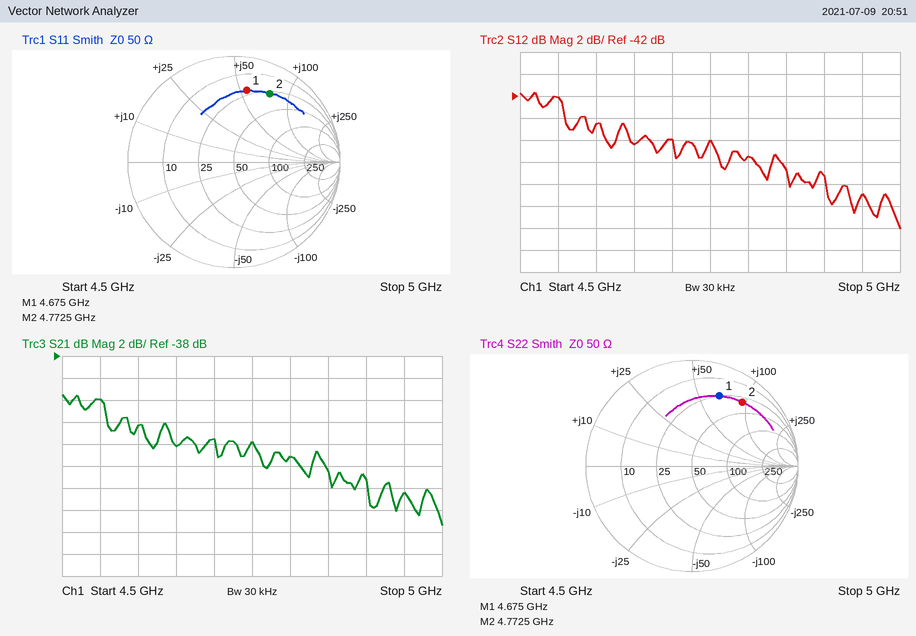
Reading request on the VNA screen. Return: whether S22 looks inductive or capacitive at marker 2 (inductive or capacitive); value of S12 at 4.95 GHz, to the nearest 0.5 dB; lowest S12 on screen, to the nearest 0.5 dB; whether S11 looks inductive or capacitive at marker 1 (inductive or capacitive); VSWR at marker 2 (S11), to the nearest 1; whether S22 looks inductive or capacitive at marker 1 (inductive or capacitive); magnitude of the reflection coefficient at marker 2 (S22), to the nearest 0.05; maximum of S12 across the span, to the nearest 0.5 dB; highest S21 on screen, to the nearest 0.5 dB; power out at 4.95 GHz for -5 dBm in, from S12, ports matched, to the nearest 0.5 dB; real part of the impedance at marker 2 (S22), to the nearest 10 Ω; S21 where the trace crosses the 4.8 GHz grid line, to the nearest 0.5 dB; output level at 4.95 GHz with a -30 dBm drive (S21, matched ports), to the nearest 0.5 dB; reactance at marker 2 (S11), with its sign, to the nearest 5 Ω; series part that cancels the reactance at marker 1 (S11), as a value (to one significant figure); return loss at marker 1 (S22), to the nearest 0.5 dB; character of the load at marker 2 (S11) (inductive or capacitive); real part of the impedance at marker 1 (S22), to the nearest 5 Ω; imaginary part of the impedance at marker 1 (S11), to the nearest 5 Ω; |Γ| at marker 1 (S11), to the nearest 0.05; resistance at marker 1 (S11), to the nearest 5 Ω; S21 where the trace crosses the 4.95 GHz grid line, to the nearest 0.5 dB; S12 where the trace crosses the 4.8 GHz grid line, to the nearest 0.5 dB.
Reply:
inductive
-51.0 dB
-54.0 dB
inductive
6
inductive
0.75
-41.5 dB
-41.5 dB
-56.0 dBm
30 Ω
-47.0 dB
-80.5 dBm
+75 Ω
600 fF
3.0 dB
inductive
25 Ω
+55 Ω
0.70
20 Ω
-50.5 dB
-47.5 dB
